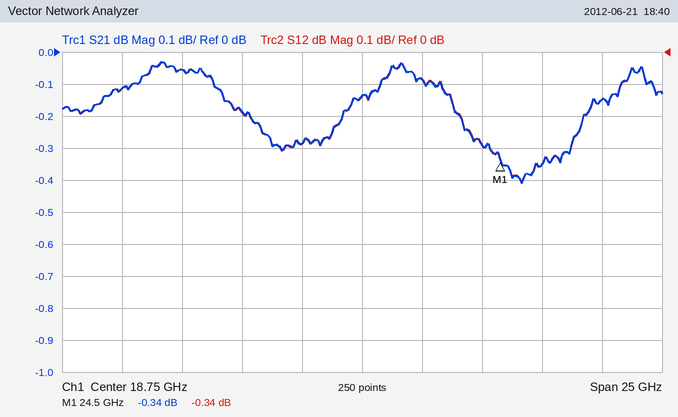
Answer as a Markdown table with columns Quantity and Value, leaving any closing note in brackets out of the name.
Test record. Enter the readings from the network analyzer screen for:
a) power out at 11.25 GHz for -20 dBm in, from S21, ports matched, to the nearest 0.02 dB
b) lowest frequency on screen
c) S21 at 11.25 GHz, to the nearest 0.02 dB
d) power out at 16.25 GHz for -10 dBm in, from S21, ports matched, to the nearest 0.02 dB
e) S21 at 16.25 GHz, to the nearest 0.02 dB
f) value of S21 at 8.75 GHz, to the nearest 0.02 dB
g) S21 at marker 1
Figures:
| Quantity | Value |
|---|---|
| power out at 11.25 GHz for -20 dBm in, from S21, ports matched, to the nearest 0.02 dB | -20.06 dBm |
| lowest frequency on screen | 6.25 GHz |
| S21 at 11.25 GHz, to the nearest 0.02 dB | -0.06 dB |
| power out at 16.25 GHz for -10 dBm in, from S21, ports matched, to the nearest 0.02 dB | -10.28 dBm |
| S21 at 16.25 GHz, to the nearest 0.02 dB | -0.28 dB |
| value of S21 at 8.75 GHz, to the nearest 0.02 dB | -0.12 dB |
| S21 at marker 1 | -0.34 dB |
